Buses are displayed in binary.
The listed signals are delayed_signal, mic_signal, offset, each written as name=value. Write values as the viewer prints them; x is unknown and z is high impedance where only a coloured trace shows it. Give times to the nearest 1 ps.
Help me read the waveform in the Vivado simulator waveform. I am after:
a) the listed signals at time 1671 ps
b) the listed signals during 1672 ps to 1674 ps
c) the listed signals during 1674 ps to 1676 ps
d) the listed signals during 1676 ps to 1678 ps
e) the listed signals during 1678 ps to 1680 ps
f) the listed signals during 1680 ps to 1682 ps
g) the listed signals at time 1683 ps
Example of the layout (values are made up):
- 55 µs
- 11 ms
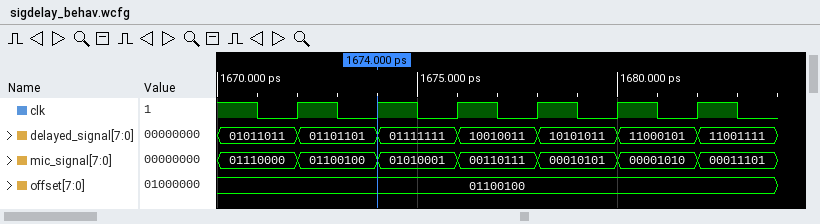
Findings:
- delayed_signal=01011011, mic_signal=01110000, offset=01100100
- delayed_signal=01101101, mic_signal=01100100, offset=01100100
- delayed_signal=01111111, mic_signal=01010001, offset=01100100
- delayed_signal=10010011, mic_signal=00110111, offset=01100100
- delayed_signal=10101011, mic_signal=00010101, offset=01100100
- delayed_signal=11000101, mic_signal=00001010, offset=01100100
- delayed_signal=11001111, mic_signal=00011101, offset=01100100
